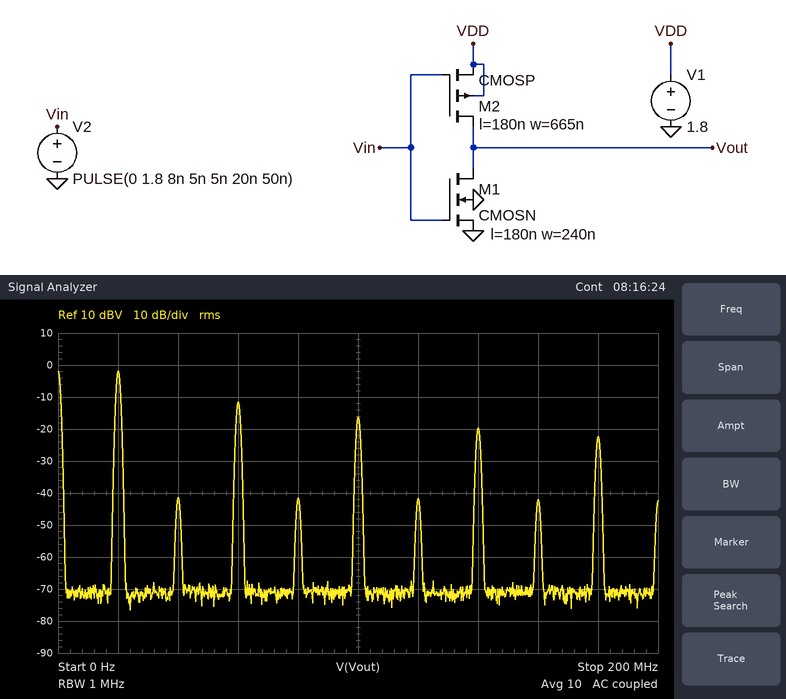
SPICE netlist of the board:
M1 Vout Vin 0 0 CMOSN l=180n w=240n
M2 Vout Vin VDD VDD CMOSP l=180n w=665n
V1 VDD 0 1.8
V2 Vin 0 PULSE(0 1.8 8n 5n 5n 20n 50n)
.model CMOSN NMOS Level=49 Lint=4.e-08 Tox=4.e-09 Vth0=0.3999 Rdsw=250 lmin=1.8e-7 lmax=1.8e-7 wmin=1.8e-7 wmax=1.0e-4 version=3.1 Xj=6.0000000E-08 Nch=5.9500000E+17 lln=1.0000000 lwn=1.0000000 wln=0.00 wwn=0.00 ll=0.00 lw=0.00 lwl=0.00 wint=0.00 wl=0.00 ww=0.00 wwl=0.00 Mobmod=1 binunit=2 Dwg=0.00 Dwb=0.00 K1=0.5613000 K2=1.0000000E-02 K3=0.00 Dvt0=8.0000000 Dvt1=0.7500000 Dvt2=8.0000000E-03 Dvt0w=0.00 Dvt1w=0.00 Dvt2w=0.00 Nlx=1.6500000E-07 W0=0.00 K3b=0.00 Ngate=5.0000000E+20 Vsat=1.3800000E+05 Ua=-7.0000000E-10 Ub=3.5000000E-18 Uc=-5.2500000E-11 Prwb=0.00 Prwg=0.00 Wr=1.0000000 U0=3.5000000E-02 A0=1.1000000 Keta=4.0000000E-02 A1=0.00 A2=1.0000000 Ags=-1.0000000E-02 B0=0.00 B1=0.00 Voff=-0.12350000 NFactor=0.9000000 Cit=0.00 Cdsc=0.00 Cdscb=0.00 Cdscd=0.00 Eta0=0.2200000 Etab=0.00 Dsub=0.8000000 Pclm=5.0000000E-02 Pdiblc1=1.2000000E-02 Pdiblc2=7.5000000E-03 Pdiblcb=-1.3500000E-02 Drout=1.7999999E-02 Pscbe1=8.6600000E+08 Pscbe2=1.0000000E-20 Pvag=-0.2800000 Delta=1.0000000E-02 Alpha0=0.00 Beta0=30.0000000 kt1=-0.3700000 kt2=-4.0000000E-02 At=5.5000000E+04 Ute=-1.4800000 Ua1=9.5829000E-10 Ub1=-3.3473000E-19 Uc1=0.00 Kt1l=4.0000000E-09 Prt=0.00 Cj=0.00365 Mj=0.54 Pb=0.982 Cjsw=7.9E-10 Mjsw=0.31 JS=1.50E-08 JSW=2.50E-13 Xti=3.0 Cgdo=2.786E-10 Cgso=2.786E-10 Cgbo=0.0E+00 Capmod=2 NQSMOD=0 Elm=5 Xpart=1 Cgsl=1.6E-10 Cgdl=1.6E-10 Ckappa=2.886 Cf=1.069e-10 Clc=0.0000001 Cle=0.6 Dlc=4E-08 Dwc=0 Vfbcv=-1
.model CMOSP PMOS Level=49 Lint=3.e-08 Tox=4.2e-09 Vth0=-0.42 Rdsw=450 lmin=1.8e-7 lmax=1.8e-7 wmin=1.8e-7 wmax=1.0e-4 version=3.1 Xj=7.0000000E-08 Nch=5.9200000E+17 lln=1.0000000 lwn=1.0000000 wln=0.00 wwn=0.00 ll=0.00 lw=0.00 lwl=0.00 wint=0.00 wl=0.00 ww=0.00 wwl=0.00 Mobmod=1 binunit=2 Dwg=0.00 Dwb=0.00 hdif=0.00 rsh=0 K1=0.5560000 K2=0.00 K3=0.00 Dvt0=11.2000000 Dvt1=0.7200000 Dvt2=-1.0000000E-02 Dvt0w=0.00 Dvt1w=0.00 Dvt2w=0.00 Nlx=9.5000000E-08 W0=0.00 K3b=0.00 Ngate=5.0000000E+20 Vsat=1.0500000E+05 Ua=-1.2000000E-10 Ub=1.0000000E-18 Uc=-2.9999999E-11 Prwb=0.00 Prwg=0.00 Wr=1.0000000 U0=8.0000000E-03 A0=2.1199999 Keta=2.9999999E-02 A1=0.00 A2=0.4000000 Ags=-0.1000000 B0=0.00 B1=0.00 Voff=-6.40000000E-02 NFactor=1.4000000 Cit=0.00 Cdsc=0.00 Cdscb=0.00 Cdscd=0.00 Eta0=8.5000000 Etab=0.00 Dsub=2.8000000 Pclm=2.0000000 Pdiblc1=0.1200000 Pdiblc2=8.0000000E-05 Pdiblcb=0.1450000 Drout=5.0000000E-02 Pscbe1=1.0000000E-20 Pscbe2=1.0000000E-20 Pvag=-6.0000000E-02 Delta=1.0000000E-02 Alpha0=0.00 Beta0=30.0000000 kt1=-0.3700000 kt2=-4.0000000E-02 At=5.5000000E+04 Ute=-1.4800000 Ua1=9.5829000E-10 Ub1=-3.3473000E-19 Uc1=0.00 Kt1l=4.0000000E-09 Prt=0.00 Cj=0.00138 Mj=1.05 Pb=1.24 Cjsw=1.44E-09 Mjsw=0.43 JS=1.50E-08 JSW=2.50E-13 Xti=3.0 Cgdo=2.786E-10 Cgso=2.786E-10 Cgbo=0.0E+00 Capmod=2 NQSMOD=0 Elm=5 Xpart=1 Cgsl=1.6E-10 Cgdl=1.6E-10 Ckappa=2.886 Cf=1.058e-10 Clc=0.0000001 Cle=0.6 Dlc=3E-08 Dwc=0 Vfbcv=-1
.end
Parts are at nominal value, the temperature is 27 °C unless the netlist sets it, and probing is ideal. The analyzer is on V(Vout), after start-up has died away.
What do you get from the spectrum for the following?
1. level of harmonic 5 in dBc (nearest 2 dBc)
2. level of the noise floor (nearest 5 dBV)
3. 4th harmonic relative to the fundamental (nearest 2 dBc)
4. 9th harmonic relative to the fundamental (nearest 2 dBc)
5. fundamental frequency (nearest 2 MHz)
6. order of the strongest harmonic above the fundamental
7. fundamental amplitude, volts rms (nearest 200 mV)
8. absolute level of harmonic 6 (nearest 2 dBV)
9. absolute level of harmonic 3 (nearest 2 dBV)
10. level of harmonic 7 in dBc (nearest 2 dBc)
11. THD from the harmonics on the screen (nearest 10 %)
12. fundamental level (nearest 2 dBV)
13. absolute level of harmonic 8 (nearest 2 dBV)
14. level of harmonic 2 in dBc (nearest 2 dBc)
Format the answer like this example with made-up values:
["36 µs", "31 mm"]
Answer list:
["-14 dBc", "-70 dBV", "-40 dBc", "-20 dBc", "20 MHz", "3", "800 mV", "-42 dBV", "-12 dBV", "-18 dBc", "40 %", "-2 dBV", "-42 dBV", "-40 dBc"]
